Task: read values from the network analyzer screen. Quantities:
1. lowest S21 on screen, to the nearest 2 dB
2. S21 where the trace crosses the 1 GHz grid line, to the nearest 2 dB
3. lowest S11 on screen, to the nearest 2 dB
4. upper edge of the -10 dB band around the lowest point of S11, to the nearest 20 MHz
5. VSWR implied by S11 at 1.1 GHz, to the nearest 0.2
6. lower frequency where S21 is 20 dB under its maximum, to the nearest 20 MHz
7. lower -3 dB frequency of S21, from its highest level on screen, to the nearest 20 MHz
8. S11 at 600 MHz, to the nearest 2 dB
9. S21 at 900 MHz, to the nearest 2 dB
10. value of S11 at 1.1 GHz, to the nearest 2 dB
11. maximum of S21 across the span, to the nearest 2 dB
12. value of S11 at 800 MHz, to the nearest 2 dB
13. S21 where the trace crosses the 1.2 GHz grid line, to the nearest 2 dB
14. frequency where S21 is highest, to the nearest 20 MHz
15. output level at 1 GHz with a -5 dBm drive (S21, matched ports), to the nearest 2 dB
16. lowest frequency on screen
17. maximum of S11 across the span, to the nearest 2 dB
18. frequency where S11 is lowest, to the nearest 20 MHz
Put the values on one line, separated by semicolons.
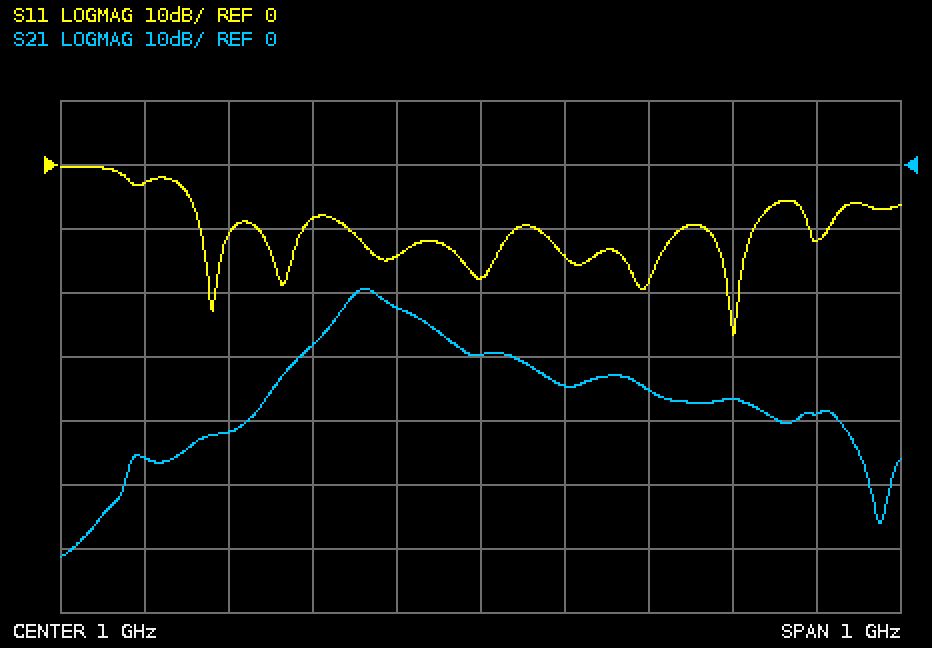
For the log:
-62 dB; -30 dB; -26 dB; 1.32 GHz; 1.4; 720 MHz; 840 MHz; -2 dB; -22 dB; -14 dB; -20 dB; -8 dB; -36 dB; 860 MHz; -34 dBm; 500 MHz; 0 dB; 1.30 GHz
